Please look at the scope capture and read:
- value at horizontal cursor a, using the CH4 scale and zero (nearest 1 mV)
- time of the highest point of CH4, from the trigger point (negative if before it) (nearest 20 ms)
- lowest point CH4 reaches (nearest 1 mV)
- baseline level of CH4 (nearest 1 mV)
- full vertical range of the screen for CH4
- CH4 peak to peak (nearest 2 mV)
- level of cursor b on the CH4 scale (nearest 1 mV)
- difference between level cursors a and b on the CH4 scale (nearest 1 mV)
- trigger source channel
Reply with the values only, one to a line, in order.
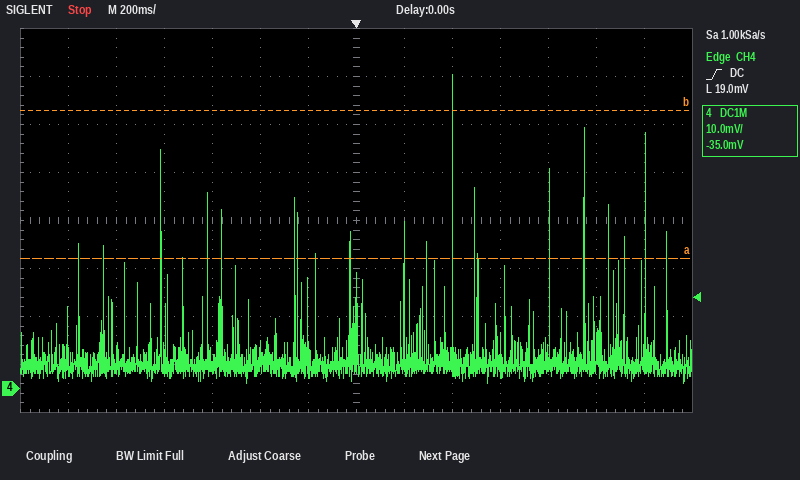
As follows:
27 mV
+400 ms
1 mV
5 mV
80 mV
64 mV
58 mV
31 mV
CH4
